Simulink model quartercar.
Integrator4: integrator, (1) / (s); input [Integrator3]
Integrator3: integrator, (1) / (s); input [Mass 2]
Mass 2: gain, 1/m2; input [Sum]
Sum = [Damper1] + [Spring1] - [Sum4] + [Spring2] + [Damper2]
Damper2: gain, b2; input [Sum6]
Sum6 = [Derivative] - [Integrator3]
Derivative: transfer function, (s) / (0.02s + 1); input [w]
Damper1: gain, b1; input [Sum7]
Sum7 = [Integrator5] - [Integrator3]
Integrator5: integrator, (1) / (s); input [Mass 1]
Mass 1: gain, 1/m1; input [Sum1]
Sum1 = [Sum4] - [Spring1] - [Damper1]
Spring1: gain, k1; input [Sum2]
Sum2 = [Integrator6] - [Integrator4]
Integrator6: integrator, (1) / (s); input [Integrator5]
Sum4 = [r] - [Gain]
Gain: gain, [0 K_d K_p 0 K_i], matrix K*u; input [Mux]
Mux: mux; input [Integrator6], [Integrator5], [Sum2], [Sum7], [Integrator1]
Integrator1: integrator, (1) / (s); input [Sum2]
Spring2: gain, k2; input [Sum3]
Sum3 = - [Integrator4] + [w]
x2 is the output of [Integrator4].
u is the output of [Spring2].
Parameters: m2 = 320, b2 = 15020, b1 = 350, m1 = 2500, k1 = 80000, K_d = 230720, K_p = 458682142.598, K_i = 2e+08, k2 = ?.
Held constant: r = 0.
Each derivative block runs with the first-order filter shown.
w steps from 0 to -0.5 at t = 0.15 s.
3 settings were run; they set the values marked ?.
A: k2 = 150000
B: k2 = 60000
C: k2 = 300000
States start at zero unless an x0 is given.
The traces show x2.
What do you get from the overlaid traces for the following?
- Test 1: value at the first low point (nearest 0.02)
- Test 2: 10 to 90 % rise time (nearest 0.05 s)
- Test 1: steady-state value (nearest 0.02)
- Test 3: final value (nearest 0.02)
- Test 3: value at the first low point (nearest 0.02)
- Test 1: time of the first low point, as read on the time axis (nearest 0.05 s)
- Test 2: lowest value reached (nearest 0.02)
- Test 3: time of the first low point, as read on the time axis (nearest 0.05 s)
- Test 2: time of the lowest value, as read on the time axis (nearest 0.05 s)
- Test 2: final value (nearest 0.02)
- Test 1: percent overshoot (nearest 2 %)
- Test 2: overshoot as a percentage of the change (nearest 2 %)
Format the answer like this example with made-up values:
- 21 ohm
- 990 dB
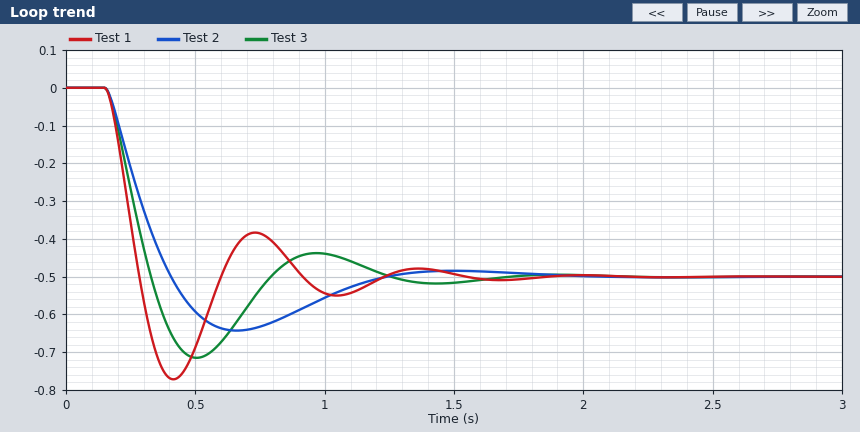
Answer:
- -0.78
- 0.20 s
- -0.50
- -0.50
- -0.72
- 0.40 s
- -0.64
- 0.50 s
- 0.65 s
- -0.50
- 54 %
- 28 %
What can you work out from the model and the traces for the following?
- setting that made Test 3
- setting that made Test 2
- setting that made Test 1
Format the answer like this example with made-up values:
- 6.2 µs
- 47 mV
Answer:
- A
- B
- C
